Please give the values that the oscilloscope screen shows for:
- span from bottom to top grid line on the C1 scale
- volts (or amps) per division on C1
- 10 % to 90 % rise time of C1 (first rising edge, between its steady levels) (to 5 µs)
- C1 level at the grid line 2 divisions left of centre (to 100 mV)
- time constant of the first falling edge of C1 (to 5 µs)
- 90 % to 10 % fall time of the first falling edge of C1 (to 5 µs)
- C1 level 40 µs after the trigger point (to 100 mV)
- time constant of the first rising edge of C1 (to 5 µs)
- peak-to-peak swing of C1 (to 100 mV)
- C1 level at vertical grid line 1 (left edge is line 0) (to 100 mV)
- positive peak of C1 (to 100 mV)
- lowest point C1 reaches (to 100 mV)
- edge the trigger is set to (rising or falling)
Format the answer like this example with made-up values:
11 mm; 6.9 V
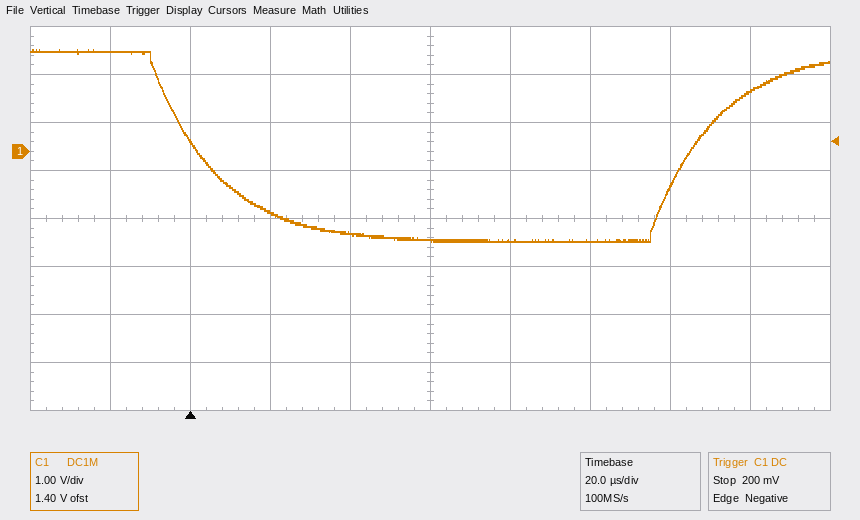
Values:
8 V; 1 V; 35 µs; -1.3 V; 15 µs; 35 µs; -1.7 V; 15 µs; 4.0 V; 2.1 V; 2.1 V; -1.9 V; falling
